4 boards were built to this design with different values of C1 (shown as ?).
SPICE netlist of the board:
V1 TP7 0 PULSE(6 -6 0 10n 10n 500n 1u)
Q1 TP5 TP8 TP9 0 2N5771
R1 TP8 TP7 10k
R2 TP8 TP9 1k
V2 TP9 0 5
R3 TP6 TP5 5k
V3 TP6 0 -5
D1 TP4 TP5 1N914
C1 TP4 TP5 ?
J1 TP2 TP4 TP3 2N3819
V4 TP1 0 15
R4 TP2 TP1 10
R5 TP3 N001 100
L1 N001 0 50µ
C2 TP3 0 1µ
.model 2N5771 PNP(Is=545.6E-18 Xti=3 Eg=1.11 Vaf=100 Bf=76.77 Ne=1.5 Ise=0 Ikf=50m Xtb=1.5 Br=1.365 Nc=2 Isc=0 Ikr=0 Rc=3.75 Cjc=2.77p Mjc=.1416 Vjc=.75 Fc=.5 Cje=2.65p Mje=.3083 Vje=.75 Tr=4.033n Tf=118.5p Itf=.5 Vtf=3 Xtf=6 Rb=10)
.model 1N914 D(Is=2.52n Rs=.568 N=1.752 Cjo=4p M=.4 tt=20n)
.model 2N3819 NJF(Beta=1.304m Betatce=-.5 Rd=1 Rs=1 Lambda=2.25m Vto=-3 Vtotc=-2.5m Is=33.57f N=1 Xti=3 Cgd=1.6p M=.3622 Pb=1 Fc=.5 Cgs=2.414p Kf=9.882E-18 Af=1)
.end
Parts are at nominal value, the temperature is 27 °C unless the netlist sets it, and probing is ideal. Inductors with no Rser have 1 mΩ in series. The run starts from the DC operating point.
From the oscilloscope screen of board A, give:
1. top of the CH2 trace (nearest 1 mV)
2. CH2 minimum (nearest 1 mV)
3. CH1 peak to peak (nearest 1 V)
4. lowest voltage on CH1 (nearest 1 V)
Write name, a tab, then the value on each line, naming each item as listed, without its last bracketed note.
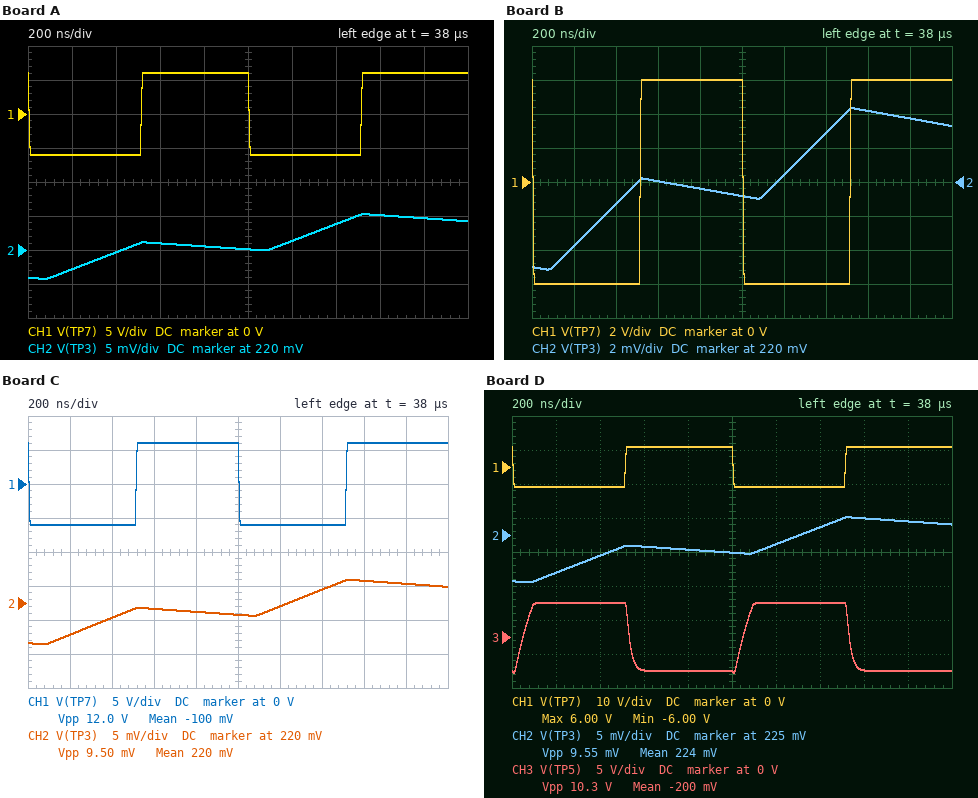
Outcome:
top of the CH2 trace	225 mV
CH2 minimum	216 mV
CH1 peak to peak	12 V
lowest voltage on CH1	-6 V
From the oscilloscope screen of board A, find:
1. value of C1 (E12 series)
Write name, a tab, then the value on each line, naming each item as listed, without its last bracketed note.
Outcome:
value of C1	560 pF
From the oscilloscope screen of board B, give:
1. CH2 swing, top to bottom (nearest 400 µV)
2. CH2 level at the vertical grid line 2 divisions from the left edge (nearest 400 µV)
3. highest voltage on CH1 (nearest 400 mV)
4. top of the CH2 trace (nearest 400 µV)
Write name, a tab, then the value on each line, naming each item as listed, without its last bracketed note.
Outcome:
CH2 swing, top to bottom	9.6 mV
CH2 level at the vertical grid line 2 divisions from the left edge	218.8 mV
highest voltage on CH1	6.0 V
top of the CH2 trace	224.4 mV
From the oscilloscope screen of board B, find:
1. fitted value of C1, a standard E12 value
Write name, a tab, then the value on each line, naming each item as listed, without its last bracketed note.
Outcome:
fitted value of C1, a standard E12 value	470 pF
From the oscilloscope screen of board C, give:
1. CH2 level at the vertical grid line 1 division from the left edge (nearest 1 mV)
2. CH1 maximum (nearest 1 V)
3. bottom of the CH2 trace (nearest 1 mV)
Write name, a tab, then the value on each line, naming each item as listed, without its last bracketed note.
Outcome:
CH2 level at the vertical grid line 1 division from the left edge	215 mV
CH1 maximum	6 V
bottom of the CH2 trace	214 mV
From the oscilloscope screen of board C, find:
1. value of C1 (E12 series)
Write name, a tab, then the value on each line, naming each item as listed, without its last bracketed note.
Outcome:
value of C1	390 pF
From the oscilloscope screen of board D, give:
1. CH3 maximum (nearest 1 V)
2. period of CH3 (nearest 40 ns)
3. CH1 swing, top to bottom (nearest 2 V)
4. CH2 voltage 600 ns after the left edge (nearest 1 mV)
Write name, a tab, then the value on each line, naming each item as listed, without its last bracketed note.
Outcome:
CH3 maximum	5 V
period of CH3	1.00 µs
CH1 swing, top to bottom	12 V
CH2 voltage 600 ns after the left edge	223 mV
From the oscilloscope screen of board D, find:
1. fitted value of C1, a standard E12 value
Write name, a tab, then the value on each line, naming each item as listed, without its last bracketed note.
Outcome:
fitted value of C1, a standard E12 value	820 pF
